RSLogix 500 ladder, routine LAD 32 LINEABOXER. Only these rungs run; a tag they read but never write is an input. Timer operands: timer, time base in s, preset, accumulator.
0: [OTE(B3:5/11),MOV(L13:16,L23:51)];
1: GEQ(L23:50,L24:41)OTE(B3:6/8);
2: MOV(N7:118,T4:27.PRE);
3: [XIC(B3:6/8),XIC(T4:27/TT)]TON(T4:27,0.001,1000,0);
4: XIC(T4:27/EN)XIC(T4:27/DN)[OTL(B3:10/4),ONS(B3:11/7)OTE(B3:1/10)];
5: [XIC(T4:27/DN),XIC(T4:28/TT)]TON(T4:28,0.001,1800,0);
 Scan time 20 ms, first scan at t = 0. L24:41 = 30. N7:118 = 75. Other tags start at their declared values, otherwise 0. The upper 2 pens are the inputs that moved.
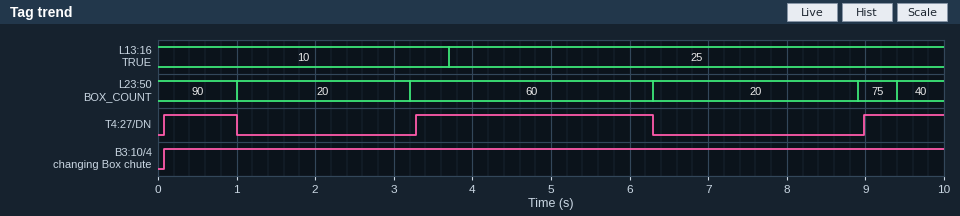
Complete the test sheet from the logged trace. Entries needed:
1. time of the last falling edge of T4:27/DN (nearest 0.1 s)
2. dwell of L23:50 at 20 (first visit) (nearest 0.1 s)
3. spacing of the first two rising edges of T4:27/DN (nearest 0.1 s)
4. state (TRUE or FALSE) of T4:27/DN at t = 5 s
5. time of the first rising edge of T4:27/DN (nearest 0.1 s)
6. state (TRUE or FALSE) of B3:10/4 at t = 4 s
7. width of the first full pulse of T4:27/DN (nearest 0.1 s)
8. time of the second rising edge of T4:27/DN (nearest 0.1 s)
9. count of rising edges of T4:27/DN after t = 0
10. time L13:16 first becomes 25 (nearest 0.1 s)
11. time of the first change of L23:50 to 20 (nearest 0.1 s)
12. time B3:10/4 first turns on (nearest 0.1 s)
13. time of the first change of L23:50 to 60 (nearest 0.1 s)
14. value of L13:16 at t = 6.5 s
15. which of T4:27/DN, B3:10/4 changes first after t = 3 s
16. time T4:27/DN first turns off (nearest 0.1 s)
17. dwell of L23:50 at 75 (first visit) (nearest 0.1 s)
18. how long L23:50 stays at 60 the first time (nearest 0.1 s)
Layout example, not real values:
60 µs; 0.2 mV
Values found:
6.3 s; 2.2 s; 3.2 s; TRUE; 0.1 s; TRUE; 0.9 s; 3.3 s; 3; 3.7 s; 1.0 s; 0.1 s; 3.2 s; 25; T4:27/DN; 1.0 s; 0.5 s; 3.1 s
